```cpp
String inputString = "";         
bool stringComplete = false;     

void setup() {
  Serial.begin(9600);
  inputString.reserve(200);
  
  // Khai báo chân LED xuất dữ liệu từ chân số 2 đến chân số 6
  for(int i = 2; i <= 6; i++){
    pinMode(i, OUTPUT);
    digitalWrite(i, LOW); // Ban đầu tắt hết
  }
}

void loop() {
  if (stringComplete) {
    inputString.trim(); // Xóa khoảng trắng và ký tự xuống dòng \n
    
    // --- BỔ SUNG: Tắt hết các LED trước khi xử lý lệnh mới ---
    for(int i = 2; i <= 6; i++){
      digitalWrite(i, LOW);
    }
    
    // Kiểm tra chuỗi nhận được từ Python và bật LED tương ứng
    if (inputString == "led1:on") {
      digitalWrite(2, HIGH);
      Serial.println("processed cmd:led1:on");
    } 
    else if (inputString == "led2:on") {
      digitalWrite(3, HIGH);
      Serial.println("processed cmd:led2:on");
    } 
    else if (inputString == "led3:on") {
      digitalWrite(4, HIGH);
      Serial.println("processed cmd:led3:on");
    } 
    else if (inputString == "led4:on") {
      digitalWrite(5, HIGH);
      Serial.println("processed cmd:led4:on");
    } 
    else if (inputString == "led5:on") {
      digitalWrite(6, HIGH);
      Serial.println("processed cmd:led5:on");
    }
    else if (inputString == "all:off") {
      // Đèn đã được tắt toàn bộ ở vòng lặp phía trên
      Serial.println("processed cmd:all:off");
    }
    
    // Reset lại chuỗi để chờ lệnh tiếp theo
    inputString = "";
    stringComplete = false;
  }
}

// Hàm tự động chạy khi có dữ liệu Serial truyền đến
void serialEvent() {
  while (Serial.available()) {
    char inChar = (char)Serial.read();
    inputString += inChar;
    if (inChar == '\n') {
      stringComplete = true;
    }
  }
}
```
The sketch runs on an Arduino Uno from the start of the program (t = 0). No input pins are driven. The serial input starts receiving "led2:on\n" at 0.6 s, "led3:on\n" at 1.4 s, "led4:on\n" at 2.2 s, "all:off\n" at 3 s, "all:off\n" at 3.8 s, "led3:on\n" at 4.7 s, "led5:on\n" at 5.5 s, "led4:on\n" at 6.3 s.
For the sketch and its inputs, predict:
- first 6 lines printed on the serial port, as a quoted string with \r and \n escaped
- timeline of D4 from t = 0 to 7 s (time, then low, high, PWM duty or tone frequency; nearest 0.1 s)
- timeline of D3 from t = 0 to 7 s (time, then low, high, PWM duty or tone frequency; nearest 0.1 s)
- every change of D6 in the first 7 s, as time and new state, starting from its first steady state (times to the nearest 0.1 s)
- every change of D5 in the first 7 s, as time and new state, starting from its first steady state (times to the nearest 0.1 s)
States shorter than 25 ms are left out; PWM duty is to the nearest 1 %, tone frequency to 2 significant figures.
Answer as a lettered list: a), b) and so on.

a) "processed cmd:led2:on\r\nprocessed cmd:led3:on\r\nprocessed cmd:led4:on\r\nprocessed cmd:all:off\r\nprocessed cmd:all:off\r\nprocessed cmd:led3:on\r\n"
b) 0 s low; 1.4 s high; 2.2 s low; 4.7 s high; 5.5 s low
c) 0 s low; 0.6 s high; 1.4 s low
d) 0 s low; 5.5 s high; 6.3 s low
e) 0 s low; 2.2 s high; 3 s low; 6.3 s high
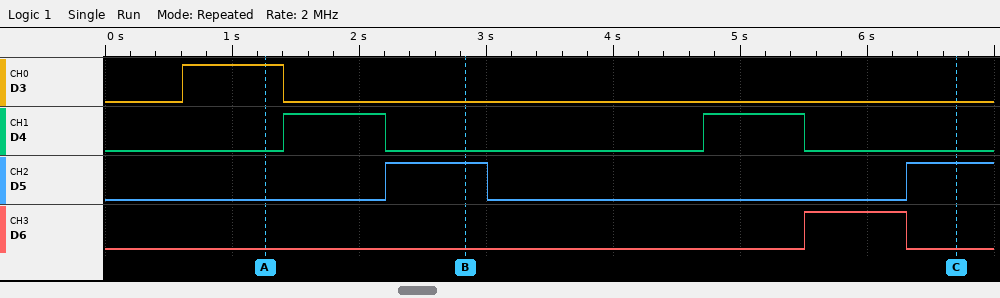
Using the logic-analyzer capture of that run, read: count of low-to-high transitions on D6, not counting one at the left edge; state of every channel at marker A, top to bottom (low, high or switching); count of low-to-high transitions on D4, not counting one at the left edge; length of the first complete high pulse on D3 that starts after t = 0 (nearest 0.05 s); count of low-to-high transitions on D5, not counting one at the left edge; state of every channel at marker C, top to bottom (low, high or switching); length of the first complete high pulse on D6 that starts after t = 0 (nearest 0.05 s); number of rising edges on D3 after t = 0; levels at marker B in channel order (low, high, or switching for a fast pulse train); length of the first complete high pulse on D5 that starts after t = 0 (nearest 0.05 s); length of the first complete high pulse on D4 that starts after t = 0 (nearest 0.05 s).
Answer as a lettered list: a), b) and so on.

a) 1
b) D3 high, D4 low, D5 low, D6 low
c) 2
d) 0.80 s
e) 2
f) D3 low, D4 low, D5 high, D6 low
g) 0.80 s
h) 1
i) D3 low, D4 low, D5 high, D6 low
j) 0.80 s
k) 0.80 s
